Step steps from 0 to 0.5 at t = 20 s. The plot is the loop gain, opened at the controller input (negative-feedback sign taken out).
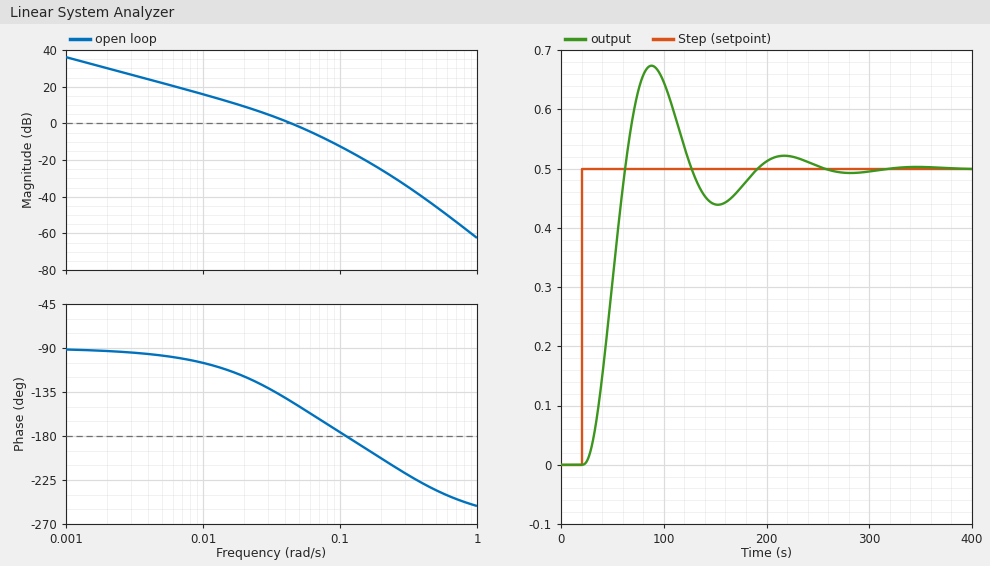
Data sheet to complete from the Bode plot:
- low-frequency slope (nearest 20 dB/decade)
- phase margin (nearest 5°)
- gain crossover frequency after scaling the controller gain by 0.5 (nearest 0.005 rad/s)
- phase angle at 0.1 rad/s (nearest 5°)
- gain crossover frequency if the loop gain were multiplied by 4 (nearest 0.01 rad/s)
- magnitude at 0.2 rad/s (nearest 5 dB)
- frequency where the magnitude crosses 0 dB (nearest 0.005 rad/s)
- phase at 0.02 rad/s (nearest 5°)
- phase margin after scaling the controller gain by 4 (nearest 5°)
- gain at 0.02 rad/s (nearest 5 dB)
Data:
-20 dB/decade
35°
0.025 rad/s
-175°
0.10 rad/s
-25 dB
0.045 rad/s
-120°
5°
10 dB
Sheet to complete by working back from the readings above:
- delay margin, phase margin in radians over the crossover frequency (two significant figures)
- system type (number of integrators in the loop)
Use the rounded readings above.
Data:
14 s
1
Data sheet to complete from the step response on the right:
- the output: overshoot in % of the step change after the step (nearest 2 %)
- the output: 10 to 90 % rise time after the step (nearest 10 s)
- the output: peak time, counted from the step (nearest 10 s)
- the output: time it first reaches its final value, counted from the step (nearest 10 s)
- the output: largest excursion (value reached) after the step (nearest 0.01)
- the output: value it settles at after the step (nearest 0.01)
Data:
34 %
30 s
70 s
40 s
0.67
0.50
